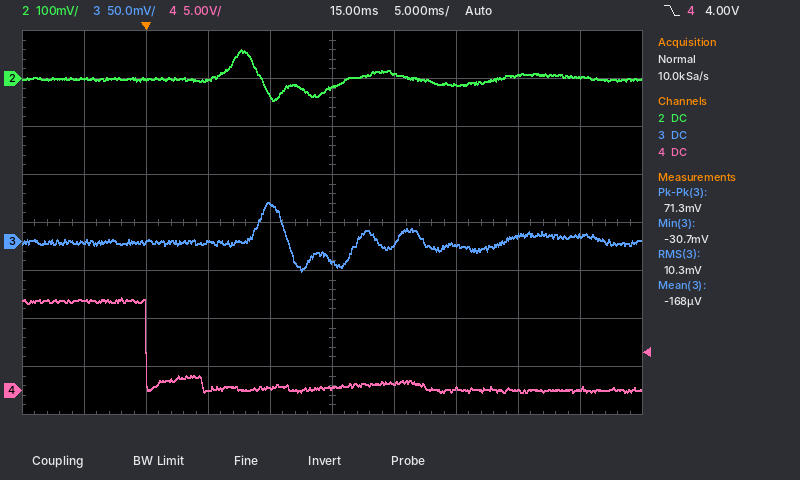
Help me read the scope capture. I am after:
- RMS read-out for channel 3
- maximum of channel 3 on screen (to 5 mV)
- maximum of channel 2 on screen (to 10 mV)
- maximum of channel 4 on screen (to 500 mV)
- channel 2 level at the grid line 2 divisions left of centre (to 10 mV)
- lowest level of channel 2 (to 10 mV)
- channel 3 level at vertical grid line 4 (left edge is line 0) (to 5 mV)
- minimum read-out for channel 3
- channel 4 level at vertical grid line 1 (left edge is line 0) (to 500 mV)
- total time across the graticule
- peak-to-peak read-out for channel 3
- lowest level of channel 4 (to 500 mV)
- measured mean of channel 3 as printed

10.3 mV
40 mV
60 mV
9.5 V
0 mV
-50 mV
40 mV
-30.7 mV
9.5 V
50 ms
71.3 mV
0.0 V
-168 µV
